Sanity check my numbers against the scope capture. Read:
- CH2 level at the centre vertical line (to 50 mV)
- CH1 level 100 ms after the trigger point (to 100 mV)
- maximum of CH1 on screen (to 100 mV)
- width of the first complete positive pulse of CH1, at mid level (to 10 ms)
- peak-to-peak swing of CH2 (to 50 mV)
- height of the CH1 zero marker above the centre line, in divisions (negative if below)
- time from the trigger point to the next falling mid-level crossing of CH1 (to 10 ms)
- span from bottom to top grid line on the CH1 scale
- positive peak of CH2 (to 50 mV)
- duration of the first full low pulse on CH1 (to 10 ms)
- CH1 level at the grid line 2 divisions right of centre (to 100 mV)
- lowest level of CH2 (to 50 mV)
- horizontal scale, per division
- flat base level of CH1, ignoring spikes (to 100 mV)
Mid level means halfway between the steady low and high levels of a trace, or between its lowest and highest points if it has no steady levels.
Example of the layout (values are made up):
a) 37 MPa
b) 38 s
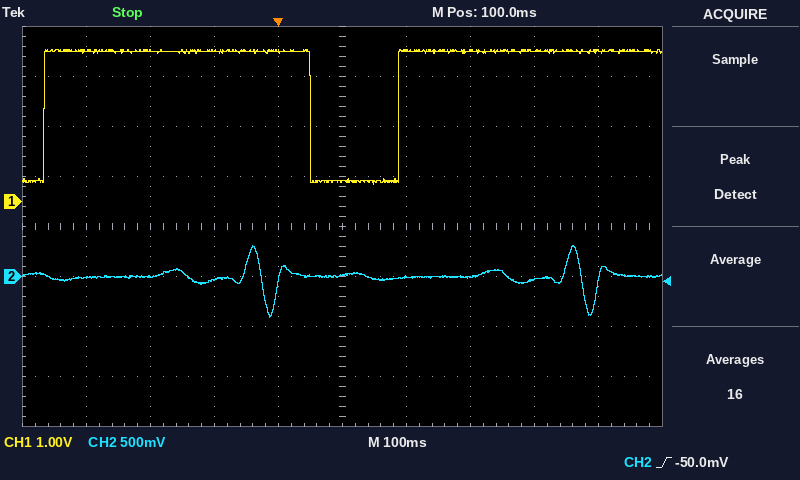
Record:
a) 0 mV
b) 400 mV
c) 3.0 V
d) 420 ms
e) 700 mV
f) +0.5 div
g) 50 ms
h) 8 V
i) 300 mV
j) 140 ms
k) 3.0 V
l) -400 mV
m) 100 ms
n) 400 mV
